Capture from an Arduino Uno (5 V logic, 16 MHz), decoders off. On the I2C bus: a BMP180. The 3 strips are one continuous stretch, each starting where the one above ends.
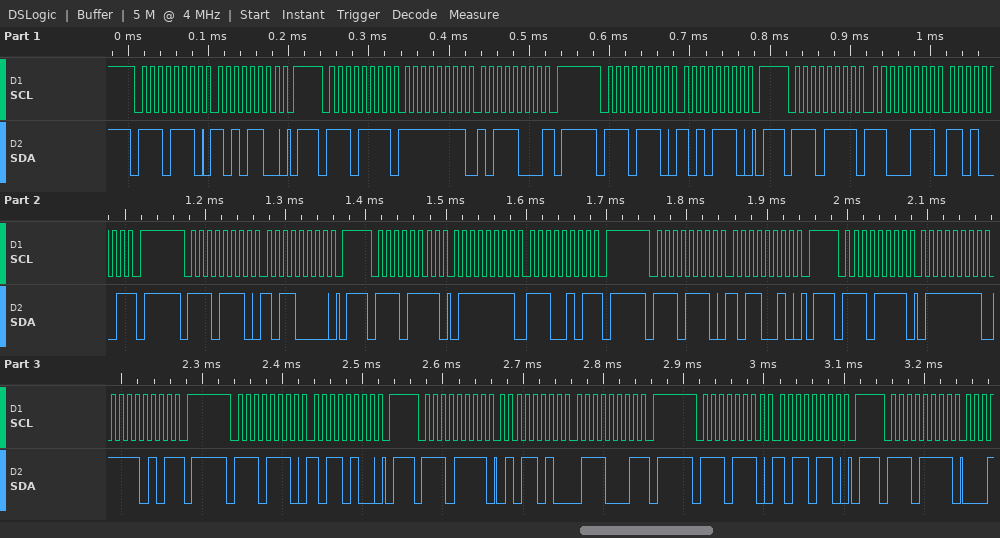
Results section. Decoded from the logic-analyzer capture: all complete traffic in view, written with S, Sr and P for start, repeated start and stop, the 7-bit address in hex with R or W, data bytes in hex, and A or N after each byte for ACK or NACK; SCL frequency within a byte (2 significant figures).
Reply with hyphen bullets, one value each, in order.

- S 77W A AC A P S 77R A FF A B8 N P S 77W A AE A P S 77R A C7 A D1 N P S 77W A B0 A P S 77R A 7F A E5 N P S 77W A B2 A P S 77R A 7F A F5 N P S 77W A B4 A P S 77R A 5A A 71 N P S 77W A B6 A P S 77R A
- 100 kHz
